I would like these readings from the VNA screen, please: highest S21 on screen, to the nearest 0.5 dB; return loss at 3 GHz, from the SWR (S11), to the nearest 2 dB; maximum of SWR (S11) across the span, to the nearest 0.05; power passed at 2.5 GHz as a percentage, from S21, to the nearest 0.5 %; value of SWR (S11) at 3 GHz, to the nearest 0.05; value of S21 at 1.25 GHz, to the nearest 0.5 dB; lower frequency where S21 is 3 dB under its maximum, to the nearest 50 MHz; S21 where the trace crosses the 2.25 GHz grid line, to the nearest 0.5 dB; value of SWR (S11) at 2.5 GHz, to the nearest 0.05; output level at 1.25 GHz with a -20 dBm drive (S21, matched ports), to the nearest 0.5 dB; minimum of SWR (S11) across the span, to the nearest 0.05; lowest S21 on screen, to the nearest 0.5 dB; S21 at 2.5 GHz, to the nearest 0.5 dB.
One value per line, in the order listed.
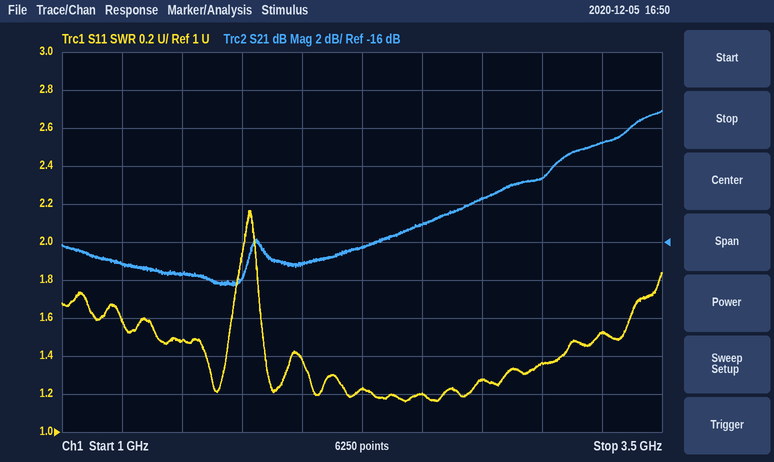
-9.0 dB
16 dB
2.15
3.0 %
1.35
-17.0 dB
3.05 GHz
-16.5 dB
1.20
-37.0 dBm
1.15
-18.5 dB
-15.0 dB
